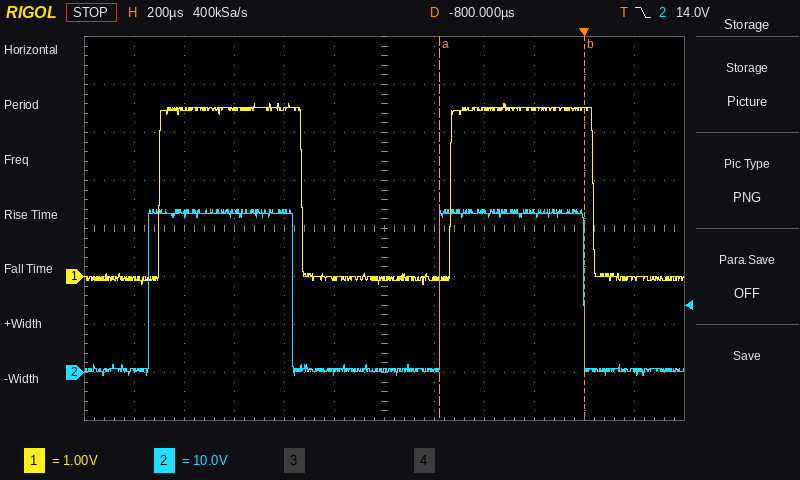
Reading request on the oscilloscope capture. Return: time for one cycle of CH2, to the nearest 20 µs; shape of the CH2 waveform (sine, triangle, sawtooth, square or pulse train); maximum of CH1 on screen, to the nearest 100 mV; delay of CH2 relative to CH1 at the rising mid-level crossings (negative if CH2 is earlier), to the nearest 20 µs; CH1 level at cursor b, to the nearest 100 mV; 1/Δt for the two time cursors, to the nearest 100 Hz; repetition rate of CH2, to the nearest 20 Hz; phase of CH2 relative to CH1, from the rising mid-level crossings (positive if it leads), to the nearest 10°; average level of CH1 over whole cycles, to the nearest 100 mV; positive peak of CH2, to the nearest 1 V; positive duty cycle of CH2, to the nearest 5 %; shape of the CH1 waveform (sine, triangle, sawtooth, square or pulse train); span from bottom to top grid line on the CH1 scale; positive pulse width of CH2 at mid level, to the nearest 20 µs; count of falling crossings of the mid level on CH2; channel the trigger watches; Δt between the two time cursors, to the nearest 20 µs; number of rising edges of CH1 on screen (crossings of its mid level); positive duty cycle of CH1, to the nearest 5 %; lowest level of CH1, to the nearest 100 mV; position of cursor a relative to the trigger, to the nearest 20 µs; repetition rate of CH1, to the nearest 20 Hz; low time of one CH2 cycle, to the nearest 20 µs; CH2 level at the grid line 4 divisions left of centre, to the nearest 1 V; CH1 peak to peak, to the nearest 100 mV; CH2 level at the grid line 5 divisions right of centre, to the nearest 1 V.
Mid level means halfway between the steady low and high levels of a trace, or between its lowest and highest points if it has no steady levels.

1.16 ms
square
3.6 V
-40 µs
3.5 V
1.7 kHz
860 Hz
+10°
1.7 V
34 V
50 %
square
8 V
580 µs
2
CH2
580 µs
2
50 %
-200 mV
-580 µs
860 Hz
580 µs
33 V
3.8 V
0 V
